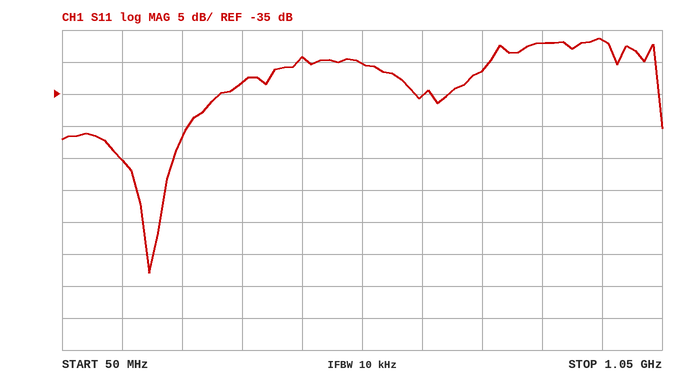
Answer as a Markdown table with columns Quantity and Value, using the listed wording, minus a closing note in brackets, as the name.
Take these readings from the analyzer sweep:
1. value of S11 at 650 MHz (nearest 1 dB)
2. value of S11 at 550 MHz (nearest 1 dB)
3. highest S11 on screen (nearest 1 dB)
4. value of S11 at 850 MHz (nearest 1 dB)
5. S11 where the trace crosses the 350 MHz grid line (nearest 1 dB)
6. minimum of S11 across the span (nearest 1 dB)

| Quantity | Value |
|---|---|
| value of S11 at 650 MHz | -35 dB |
| value of S11 at 550 MHz | -30 dB |
| highest S11 on screen | -26 dB |
| value of S11 at 850 MHz | -27 dB |
| S11 where the trace crosses the 350 MHz grid line | -33 dB |
| minimum of S11 across the span | -63 dB |
